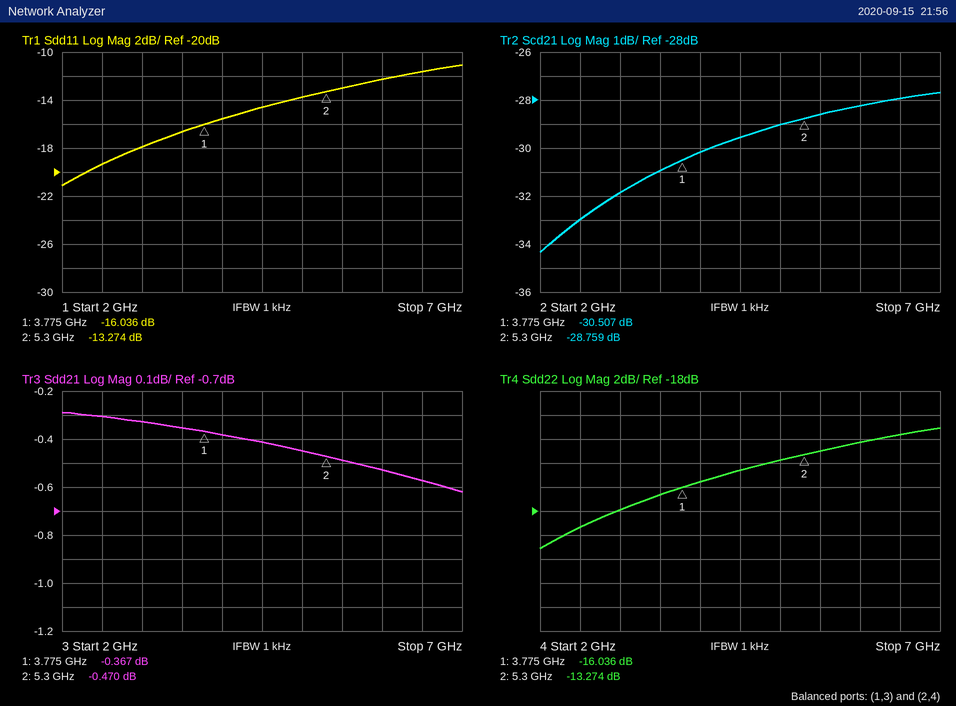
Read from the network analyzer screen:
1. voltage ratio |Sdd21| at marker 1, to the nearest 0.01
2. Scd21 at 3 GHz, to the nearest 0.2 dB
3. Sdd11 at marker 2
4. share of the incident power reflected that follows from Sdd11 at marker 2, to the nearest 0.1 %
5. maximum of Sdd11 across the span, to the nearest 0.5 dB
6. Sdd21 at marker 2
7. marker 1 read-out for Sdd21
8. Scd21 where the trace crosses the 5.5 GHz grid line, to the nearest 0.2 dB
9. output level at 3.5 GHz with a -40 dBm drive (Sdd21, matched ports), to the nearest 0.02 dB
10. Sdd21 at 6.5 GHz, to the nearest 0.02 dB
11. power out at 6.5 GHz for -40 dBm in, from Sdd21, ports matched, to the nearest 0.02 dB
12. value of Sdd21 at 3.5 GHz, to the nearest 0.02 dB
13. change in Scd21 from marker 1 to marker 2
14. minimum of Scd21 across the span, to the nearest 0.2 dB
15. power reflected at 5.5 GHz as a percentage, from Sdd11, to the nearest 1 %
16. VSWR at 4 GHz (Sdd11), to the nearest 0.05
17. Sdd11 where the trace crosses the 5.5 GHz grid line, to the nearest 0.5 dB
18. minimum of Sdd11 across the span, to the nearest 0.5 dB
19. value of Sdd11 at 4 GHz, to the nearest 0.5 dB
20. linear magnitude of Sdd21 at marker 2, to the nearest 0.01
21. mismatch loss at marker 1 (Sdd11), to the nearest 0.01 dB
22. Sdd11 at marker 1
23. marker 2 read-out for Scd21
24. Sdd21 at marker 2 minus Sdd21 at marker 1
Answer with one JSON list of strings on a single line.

["0.96", "-31.8 dB", "-13.274 dB", "4.7 %", "-11.0 dB", "-0.470 dB", "-0.367 dB", "-28.6 dB", "-40.36 dBm", "-0.58 dB", "-40.58 dBm", "-0.36 dB", "1.748 dB", "-34.4 dB", "5 %", "1.40", "-13.0 dB", "-21.0 dB", "-15.5 dB", "0.95", "0.11 dB", "-16.036 dB", "-28.759 dB", "-0.103 dB"]
